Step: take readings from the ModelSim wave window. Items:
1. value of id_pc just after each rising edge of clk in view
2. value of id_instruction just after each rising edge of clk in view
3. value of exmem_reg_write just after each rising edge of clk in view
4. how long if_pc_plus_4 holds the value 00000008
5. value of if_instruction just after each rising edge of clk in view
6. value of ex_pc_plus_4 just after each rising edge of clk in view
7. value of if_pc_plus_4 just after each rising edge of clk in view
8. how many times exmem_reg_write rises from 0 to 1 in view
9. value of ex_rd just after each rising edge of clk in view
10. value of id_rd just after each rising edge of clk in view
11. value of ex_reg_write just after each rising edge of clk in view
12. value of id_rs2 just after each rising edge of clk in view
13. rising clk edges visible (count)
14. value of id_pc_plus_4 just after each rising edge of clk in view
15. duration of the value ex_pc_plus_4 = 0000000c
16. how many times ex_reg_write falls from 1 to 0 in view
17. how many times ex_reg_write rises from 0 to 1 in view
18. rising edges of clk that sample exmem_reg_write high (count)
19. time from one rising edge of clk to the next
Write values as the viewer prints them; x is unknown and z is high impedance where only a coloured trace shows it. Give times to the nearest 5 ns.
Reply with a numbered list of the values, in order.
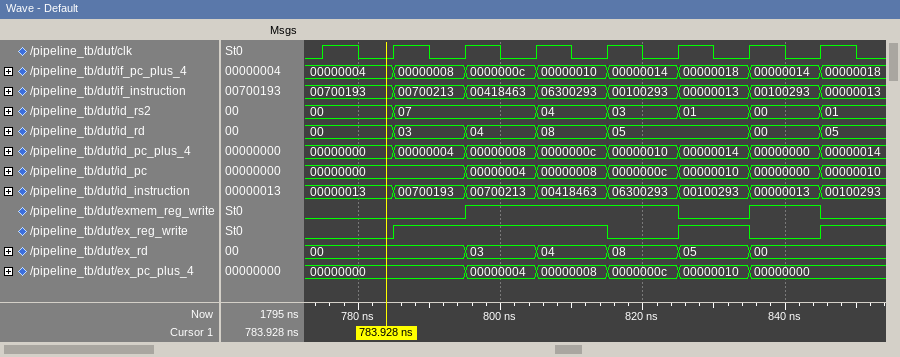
1. 00000000, 00000000, 00000004, 00000008, 0000000c, 00000010, 00000000, 00000010
2. 00000013, 00700193, 00700213, 00418463, 06300293, 00100293, 00000013, 00100293
3. 0 0 1 1 1 0 1 0
4. 10 ns
5. 00700193, 00700213, 00418463, 06300293, 00100293, 00000013, 00100293, 00000013
6. 00000000, 00000000, 00000004, 00000008, 0000000c, 00000010, 00000000, 00000000
7. 00000004, 00000008, 0000000c, 00000010, 00000014, 00000018, 00000014, 00000018
8. 2
9. 00, 00, 03, 04, 08, 05, 00, 00
10. 00, 03, 04, 08, 05, 05, 00, 05
11. 0 1 1 1 0 1 0 1
12. 00, 07, 07, 04, 03, 01, 00, 01
13. 8
14. 00000000, 00000004, 00000008, 0000000c, 00000010, 00000014, 00000000, 00000014
15. 10 ns
16. 2
17. 3
18. 4
19. 10 ns
